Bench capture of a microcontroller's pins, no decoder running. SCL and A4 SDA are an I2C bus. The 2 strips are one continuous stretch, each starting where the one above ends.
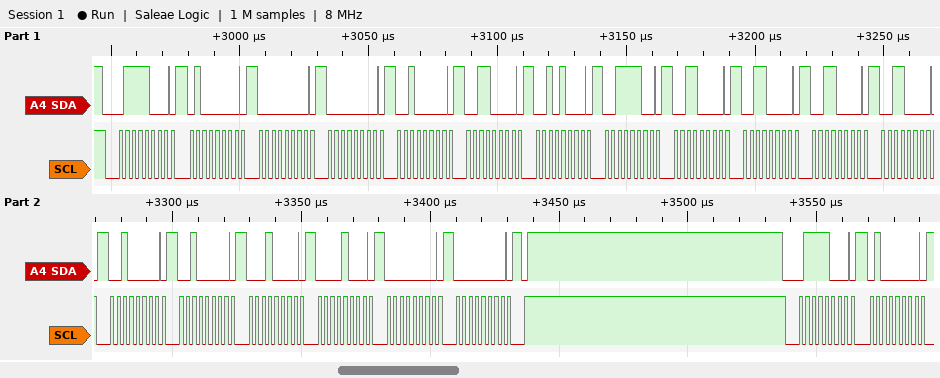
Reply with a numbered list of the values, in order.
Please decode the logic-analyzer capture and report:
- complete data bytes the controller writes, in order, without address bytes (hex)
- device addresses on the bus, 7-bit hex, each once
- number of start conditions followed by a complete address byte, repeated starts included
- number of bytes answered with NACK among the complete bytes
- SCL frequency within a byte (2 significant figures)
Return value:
1. 40 00 00 20 30 28 3C 30 30 30 30 20 20 10 08 00 00 40
2. 0x3C
3. 2
4. 0
5. 400 kHz
